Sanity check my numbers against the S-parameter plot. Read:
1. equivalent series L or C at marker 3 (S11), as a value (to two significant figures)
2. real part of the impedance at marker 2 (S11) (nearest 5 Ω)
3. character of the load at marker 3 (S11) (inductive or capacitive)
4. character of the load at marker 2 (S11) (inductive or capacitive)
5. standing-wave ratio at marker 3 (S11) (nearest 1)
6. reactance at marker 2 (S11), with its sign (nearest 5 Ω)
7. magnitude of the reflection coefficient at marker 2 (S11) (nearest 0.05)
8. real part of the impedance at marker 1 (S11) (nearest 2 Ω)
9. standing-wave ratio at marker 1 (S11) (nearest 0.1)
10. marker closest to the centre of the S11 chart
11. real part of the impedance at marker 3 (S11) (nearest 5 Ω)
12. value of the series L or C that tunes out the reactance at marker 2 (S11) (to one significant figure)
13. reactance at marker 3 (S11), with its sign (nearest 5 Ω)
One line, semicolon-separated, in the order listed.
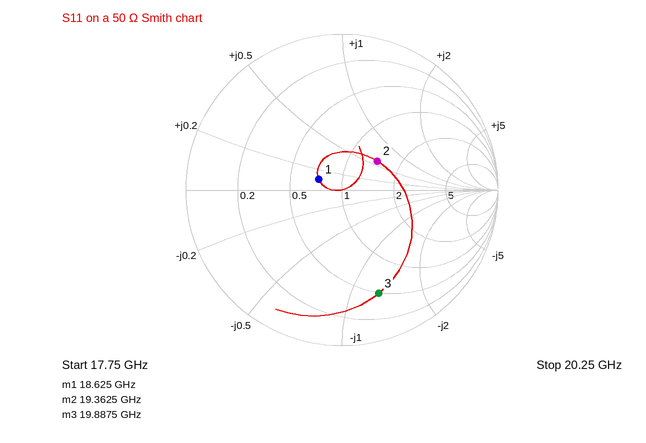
120 fF; 70 Ω; capacitive; inductive; 6; +30 Ω; 0.30; 36 Ω; 1.4; marker 1; 25 Ω; 300 fF; -65 Ω
